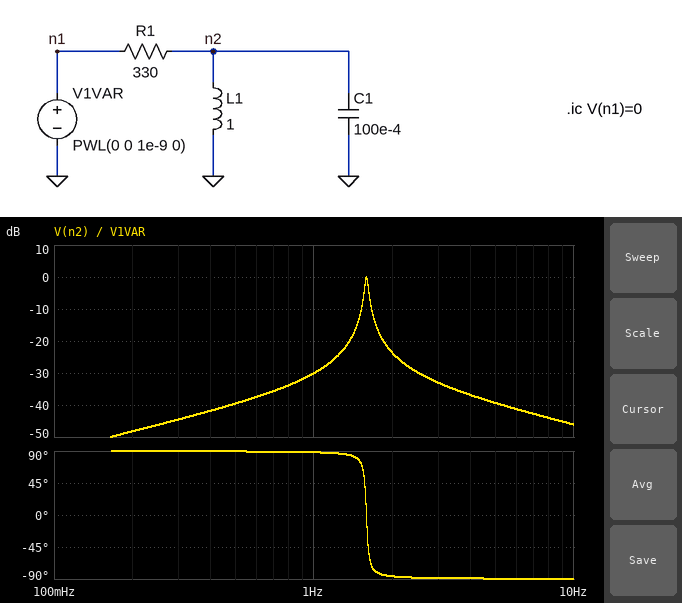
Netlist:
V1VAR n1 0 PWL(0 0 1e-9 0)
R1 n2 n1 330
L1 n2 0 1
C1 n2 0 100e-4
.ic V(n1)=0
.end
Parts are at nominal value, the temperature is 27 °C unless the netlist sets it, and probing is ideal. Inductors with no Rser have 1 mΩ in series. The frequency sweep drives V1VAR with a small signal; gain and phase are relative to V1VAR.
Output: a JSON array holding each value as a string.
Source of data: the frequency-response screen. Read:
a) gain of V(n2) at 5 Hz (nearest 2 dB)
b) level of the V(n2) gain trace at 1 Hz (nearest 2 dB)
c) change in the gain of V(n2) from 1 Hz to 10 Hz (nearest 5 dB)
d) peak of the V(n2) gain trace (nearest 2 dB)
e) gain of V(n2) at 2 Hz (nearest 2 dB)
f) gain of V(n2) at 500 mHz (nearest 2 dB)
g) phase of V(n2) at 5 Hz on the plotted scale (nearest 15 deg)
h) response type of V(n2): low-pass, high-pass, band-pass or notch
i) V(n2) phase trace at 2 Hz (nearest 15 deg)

["-40 dB", "-30 dB", "-15 dB", "0 dB", "-24 dB", "-40 dB", "-90 deg", "band-pass", "-90 deg"]
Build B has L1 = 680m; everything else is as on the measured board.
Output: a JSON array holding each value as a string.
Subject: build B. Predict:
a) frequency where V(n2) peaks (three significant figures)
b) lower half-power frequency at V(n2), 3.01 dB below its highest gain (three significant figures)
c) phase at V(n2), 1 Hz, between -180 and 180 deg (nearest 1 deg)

["1.93 Hz", "1.91 Hz", "89 deg"]
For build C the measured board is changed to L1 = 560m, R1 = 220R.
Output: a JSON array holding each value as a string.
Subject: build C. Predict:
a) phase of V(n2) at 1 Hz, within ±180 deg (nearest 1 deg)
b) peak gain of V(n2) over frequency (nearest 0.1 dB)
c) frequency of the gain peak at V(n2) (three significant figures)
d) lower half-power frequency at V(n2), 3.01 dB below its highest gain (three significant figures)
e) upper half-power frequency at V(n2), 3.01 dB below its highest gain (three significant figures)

["89 deg", "0 dB", "2.13 Hz", "2.09 Hz", "2.16 Hz"]
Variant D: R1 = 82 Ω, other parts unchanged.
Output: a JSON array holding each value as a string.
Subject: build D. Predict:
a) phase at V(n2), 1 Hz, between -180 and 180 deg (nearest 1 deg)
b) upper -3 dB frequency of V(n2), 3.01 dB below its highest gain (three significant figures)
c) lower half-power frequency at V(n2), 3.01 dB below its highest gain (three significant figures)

["83 deg", "1.69 Hz", "1.50 Hz"]
